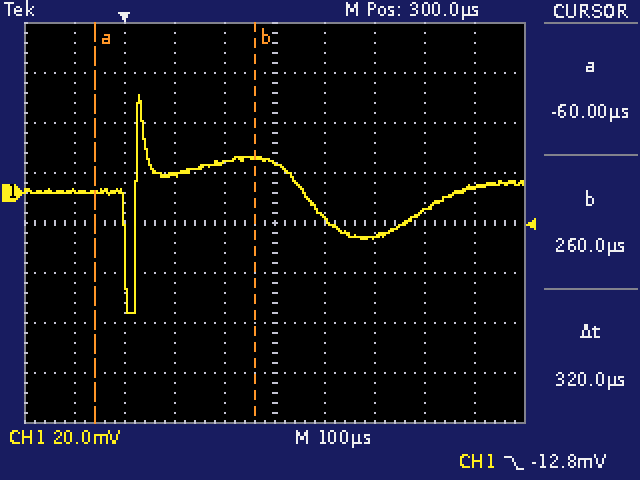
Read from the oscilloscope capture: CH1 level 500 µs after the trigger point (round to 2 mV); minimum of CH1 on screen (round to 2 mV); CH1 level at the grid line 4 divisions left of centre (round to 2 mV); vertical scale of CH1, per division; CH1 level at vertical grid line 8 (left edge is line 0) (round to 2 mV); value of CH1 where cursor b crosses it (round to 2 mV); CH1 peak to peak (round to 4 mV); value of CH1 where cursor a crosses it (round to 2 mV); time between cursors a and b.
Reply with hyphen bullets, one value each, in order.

- -18 mV
- -48 mV
- 0 mV
- 20 mV
- -8 mV
- 14 mV
- 88 mV
- 0 mV
- 320 µs
